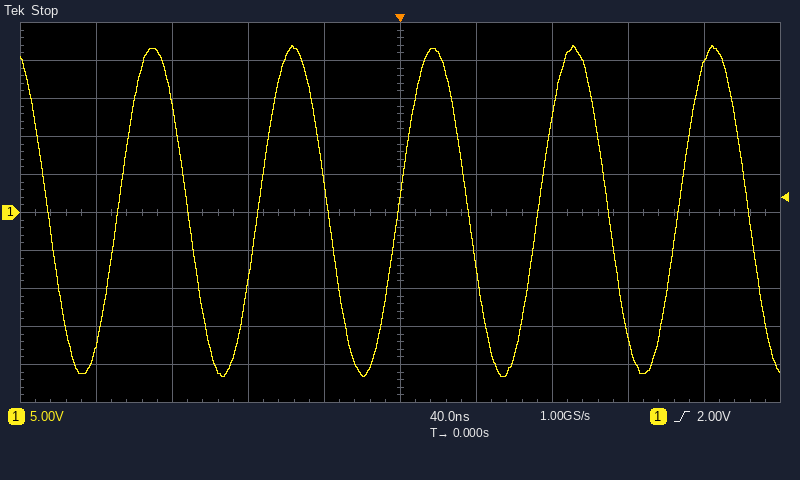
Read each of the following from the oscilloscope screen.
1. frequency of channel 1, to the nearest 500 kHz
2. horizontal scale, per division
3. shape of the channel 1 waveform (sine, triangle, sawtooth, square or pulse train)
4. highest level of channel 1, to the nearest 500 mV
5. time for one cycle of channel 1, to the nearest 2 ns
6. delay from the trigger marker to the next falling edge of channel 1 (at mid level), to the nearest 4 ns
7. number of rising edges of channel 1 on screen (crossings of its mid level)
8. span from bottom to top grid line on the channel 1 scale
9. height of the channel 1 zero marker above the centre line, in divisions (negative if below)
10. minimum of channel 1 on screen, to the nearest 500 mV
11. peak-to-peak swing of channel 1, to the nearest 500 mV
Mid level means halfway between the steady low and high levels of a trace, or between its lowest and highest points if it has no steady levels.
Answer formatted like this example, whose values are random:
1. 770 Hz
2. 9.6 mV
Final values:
1. 13.5 MHz
2. 40 ns
3. sine
4. 22.0 V
5. 74 ns
6. 36 ns
7. 5
8. 50 V
9. 0.0 div
10. -21.5 V
11. 43.5 V
